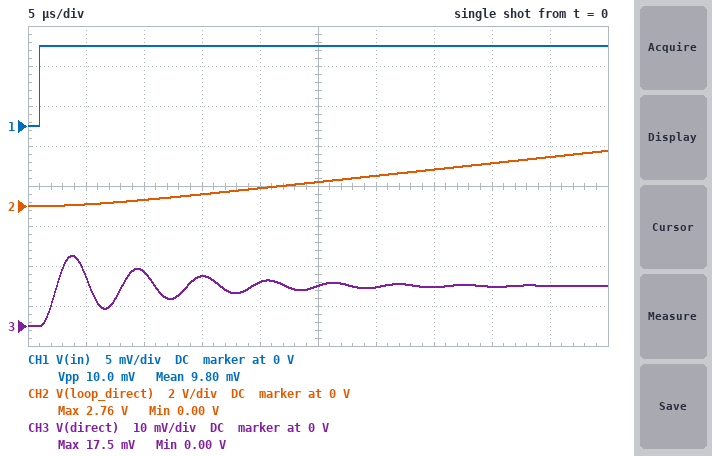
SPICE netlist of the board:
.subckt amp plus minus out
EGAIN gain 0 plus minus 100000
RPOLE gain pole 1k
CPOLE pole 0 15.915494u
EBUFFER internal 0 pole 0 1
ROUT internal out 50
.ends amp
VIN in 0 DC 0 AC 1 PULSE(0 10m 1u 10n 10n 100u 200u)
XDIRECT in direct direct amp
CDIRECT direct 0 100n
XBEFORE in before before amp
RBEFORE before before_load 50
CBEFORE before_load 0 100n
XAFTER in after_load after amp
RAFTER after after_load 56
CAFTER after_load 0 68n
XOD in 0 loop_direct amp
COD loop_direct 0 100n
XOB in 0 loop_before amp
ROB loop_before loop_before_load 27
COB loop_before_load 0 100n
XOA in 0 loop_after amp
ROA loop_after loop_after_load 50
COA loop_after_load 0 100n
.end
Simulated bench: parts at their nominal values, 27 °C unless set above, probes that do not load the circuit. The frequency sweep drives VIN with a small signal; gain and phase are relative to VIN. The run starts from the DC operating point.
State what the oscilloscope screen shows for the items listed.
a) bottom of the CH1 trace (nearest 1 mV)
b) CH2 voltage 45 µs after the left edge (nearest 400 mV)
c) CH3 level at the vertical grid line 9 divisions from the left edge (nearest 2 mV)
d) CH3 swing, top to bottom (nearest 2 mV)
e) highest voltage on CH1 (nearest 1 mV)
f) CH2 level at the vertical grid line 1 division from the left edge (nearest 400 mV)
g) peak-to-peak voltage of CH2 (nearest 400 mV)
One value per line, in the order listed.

0 V
2.4 V
10 mV
18 mV
10 mV
0 V
2.8 V
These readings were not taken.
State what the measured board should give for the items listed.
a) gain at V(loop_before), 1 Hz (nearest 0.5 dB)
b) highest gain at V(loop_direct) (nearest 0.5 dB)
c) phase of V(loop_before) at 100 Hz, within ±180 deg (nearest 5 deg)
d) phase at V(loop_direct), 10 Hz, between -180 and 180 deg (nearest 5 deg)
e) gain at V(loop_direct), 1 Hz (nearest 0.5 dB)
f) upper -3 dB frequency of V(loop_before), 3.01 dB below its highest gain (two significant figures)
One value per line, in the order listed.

100.0 dB
100.0 dB
-85 deg
-45 deg
100.0 dB
10 Hz
